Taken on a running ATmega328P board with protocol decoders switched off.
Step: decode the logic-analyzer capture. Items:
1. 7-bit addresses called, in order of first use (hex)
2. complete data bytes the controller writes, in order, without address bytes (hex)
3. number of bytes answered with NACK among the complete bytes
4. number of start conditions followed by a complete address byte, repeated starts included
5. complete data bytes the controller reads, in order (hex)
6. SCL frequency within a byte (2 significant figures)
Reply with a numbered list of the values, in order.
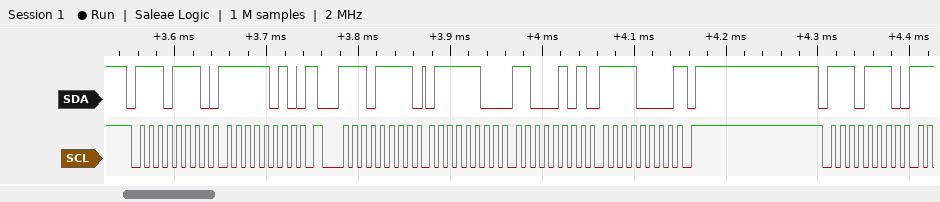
1. 0x77
2. FA
3. 1
4. 3
5. 7C C5 F0
6. 100 kHz
